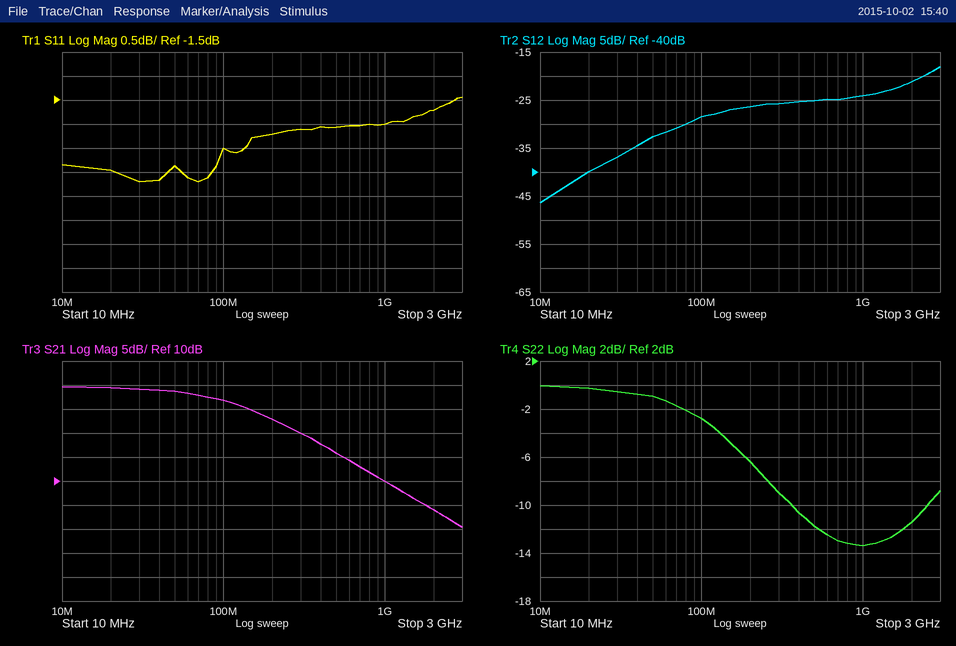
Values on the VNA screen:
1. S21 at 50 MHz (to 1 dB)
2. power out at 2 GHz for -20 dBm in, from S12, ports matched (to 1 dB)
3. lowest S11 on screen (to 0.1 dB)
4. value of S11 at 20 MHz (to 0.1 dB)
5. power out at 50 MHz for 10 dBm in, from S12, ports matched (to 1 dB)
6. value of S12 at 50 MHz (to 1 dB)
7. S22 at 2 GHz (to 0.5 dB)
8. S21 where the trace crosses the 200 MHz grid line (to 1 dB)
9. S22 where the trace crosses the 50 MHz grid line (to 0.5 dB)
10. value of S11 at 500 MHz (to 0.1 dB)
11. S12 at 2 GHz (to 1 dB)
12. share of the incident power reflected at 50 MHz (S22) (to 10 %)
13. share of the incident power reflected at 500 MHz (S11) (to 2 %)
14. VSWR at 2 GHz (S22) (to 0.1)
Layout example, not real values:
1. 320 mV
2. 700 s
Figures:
1. 29 dB
2. -41 dBm
3. -3.2 dB
4. -3.0 dB
5. -23 dBm
6. -33 dB
7. -11.5 dB
8. 23 dB
9. -1.0 dB
10. -2.1 dB
11. -21 dB
12. 80 %
13. 62 %
14. 1.7
